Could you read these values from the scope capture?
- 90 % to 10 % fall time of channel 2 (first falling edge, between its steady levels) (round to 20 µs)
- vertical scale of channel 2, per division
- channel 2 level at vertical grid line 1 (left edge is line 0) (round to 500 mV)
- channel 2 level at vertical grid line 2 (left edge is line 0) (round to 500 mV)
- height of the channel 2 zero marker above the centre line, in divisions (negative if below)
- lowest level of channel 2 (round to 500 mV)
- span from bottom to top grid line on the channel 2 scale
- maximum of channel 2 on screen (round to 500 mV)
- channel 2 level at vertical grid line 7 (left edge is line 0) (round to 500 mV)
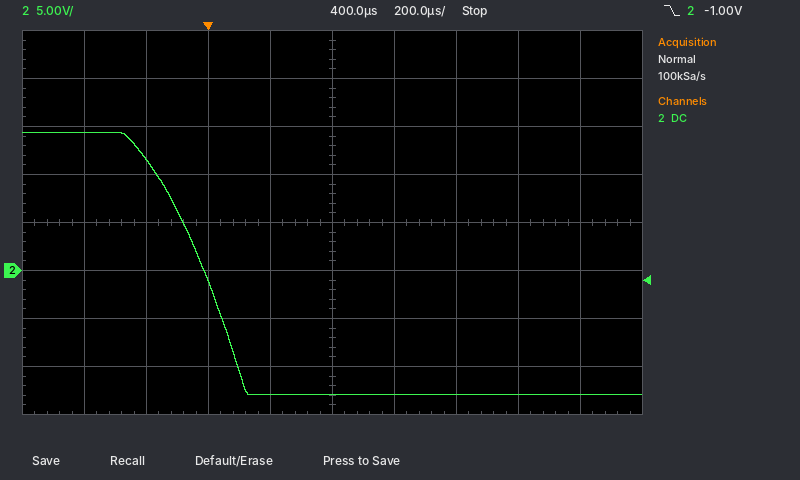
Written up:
300 µs
5 V
14.5 V
11.5 V
-1.0 div
-13.0 V
40 V
14.5 V
-13.0 V
